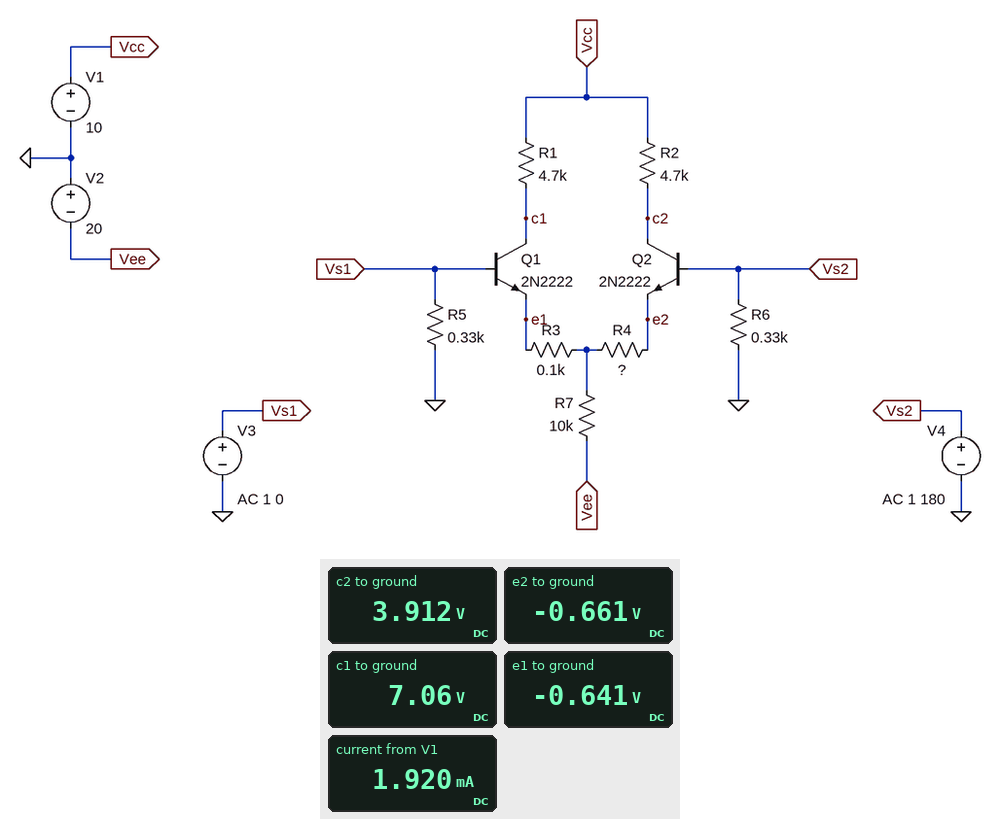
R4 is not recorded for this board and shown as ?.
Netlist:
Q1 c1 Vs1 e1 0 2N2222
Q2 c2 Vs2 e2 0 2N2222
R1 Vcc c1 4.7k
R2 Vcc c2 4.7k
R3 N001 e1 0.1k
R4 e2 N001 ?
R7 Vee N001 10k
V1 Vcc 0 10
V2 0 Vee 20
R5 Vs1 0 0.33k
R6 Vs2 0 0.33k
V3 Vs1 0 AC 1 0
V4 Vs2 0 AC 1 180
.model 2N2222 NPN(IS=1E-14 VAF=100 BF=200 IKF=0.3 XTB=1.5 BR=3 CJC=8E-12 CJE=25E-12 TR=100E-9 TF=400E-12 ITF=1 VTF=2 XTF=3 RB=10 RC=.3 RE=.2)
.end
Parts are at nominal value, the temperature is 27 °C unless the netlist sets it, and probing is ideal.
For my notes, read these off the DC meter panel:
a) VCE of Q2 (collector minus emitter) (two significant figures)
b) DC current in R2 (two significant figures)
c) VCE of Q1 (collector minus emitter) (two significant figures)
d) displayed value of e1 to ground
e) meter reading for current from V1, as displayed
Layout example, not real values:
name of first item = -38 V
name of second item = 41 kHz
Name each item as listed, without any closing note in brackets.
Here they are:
VCE of Q2 (collector minus emitter) = 4.6 V
DC current in R2 = 1.3 mA
VCE of Q1 (collector minus emitter) = 7.7 V
displayed value of e1 to ground = -0.641 V
meter reading for current from V1, as displayed = 1.920 mA
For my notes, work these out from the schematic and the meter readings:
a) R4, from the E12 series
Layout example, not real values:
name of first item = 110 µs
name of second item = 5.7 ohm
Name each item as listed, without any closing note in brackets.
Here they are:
R4, from the E12 series = 33 Ω
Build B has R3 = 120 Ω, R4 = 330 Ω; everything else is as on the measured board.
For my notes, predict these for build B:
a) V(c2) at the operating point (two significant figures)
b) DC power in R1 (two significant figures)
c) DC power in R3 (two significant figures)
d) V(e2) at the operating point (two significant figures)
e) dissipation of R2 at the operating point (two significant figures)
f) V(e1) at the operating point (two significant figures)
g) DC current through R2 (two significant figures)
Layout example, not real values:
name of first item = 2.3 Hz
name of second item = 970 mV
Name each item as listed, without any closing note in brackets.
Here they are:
V(c2) at the operating point = 7.4 V
DC power in R1 = 8.5 mW
DC power in R3 = 220 µW
V(e2) at the operating point = -640 mV
dissipation of R2 at the operating point = 1.5 mW
V(e1) at the operating point = -660 mV
DC current through R2 = 560 µA
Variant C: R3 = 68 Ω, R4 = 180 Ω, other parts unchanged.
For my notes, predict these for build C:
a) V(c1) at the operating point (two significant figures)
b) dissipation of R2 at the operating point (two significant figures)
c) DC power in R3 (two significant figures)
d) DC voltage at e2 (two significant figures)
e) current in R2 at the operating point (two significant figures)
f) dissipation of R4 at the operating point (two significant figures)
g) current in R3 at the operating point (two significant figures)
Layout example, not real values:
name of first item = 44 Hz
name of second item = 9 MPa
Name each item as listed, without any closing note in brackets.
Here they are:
V(c1) at the operating point = 3.9 V
dissipation of R2 at the operating point = 1.7 mW
DC power in R3 = 120 µW
DC voltage at e2 = -640 mV
current in R2 at the operating point = 610 µA
dissipation of R4 at the operating point = 67 µW
current in R3 at the operating point = 1.3 mA
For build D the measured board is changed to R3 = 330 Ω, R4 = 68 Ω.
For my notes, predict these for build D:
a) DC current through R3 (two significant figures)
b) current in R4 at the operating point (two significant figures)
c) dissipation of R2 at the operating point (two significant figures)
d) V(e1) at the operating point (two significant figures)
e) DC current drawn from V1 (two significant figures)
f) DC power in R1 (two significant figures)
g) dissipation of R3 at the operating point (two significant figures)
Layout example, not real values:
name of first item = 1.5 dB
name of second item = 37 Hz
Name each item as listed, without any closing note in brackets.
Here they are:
DC current through R3 = 420 µA
current in R4 at the operating point = 1.5 mA
dissipation of R2 at the operating point = 11 mW
V(e1) at the operating point = -630 mV
DC current drawn from V1 = 1.9 mA
DC power in R1 = 810 µW
dissipation of R3 at the operating point = 57 µW
